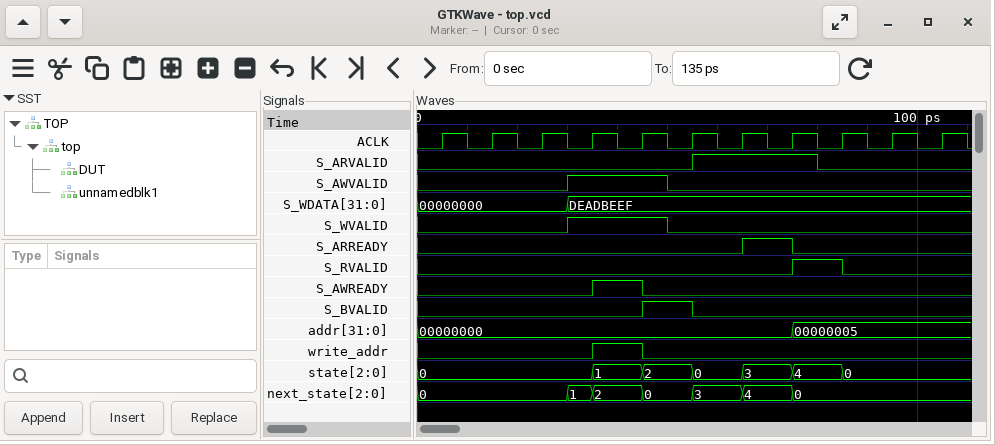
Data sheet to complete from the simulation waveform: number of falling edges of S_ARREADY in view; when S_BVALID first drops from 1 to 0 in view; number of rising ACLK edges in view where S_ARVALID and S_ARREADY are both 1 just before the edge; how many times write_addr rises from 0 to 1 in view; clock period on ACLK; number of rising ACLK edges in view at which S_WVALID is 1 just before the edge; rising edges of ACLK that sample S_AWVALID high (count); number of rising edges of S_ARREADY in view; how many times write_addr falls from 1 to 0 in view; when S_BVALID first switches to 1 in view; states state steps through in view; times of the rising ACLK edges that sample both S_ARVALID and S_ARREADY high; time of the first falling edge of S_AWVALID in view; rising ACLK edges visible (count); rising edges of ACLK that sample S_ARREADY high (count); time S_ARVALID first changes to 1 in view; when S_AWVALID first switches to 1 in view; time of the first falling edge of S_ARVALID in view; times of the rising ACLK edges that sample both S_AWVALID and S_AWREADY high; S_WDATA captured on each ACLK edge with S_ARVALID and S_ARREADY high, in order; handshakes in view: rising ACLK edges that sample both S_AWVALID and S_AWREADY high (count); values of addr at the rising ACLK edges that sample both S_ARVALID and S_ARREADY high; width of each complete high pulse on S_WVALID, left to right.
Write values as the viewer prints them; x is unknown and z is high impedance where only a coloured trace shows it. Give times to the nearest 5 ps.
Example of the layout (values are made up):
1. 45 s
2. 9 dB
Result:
1. 1
2. 55 ps
3. 1
4. 1
5. 10 ps
6. 2
7. 2
8. 1
9. 1
10. 45 ps
11. 0, 1, 2, 0, 3, 4, 0
12. 75 ps
13. 50 ps
14. 11
15. 1
16. 55 ps
17. 30 ps
18. 80 ps
19. 45 ps
20. DEADBEEF
21. 1
22. 00000000
23. 20 ps
